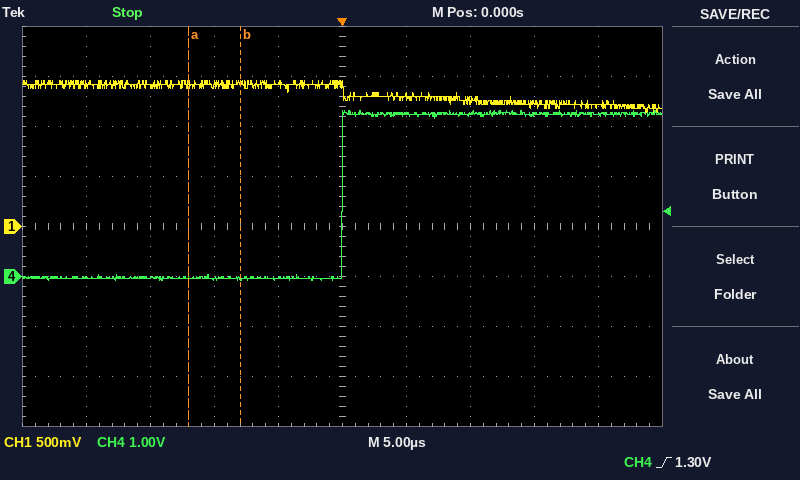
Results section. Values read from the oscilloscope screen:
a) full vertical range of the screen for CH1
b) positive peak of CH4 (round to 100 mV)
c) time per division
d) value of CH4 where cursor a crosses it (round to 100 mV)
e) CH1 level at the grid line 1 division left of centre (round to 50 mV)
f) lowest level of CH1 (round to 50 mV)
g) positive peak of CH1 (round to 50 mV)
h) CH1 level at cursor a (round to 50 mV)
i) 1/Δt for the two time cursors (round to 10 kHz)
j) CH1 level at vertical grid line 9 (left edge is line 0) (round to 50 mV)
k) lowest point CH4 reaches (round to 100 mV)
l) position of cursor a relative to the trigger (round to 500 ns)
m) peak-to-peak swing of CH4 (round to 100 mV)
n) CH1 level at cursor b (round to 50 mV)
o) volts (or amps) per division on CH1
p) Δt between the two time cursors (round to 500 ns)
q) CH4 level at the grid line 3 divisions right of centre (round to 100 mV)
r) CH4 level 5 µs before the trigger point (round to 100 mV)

4 V
3.3 V
5 µs
0.0 V
1.40 V
1.15 V
1.45 V
1.40 V
250 kHz
1.20 V
-100 mV
-12.0 µs
3.4 V
1.45 V
500 mV
4.0 µs
3.2 V
0.0 V
